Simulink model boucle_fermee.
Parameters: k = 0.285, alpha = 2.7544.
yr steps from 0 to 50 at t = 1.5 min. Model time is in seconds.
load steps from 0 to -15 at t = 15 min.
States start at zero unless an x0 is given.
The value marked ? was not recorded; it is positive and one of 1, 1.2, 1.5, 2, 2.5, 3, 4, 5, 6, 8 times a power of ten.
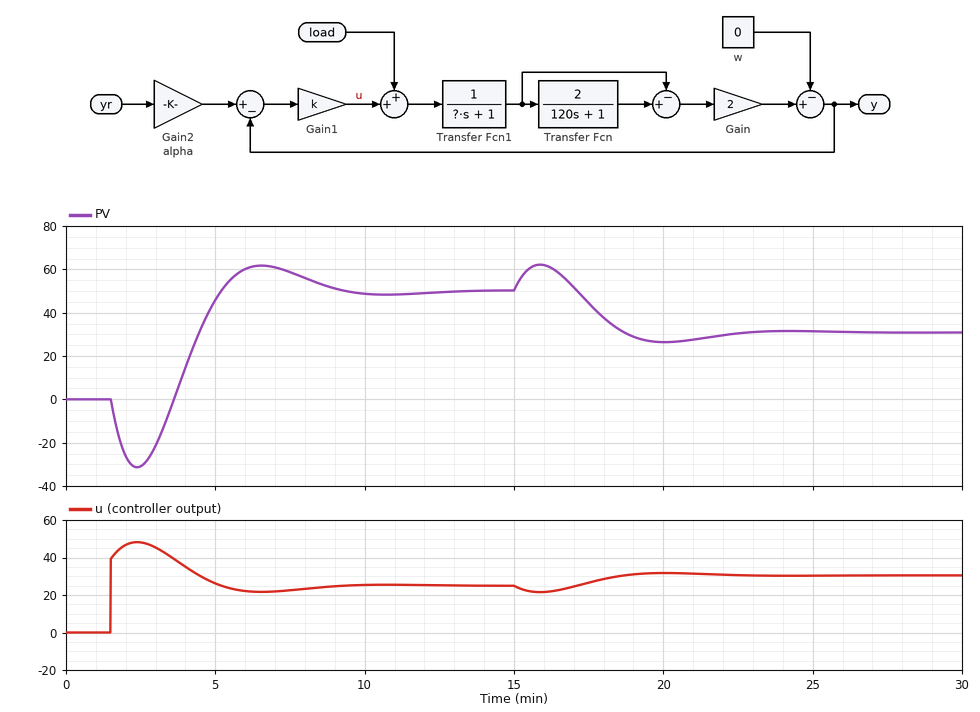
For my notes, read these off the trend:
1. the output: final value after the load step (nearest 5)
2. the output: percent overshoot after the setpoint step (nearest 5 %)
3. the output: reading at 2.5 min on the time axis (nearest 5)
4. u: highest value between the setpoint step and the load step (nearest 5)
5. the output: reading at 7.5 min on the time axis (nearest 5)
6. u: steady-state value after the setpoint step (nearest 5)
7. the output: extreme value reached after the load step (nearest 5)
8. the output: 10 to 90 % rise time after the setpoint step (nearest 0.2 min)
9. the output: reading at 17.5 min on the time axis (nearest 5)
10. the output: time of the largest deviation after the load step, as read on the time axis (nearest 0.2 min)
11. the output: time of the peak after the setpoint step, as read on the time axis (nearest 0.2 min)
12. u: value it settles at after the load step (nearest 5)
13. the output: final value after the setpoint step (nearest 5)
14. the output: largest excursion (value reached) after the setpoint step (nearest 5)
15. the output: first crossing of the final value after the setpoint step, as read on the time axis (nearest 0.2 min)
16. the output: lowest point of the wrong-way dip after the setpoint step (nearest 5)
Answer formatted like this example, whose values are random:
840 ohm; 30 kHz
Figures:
30; 25 %; -30; 50; 60; 25; 25; 1.2 min; 45; 20.0 min; 6.6 min; 30; 50; 60; 5.2 min; -30
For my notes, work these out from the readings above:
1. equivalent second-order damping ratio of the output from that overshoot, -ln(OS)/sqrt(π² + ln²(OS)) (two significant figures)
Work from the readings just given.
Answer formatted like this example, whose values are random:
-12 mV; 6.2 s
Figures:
0.40
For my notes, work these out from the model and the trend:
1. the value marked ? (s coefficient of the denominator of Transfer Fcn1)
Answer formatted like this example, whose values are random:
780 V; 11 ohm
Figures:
60
